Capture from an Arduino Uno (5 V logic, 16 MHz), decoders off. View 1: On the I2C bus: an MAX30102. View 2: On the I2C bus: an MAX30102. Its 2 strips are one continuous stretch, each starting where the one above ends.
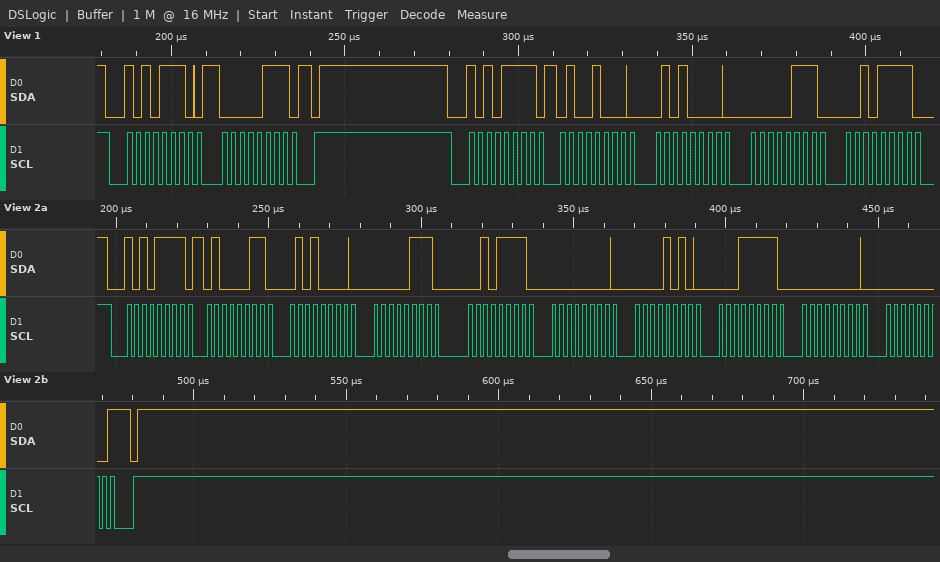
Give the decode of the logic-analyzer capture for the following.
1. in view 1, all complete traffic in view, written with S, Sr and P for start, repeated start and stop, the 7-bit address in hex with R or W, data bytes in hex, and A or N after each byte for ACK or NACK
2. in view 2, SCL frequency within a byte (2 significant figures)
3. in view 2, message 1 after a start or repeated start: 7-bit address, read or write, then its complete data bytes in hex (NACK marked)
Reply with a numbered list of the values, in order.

1. S 57W A 07 A P S 57R A 48 A 50 A 07 A 2F A
2. 400 kHz
3. 0x57 read: 43 50 07 2F 00 0A 1F 00 00 NACK
